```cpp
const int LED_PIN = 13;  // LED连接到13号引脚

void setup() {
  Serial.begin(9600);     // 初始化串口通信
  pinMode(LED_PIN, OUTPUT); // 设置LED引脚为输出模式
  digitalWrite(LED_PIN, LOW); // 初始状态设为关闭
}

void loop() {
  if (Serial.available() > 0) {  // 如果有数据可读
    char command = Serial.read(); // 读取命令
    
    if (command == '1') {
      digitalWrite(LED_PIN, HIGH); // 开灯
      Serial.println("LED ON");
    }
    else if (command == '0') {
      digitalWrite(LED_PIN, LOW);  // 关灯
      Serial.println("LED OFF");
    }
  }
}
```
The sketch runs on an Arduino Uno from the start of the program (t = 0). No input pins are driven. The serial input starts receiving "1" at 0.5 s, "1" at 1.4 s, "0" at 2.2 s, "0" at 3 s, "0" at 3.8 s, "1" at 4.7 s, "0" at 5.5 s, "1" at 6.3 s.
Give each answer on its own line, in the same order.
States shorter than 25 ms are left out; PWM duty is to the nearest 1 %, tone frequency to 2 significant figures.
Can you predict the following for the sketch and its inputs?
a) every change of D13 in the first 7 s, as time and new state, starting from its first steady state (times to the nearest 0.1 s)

0 s low; 0.5 s high; 2.2 s low; 4.7 s high; 5.5 s low; 6.3 s high
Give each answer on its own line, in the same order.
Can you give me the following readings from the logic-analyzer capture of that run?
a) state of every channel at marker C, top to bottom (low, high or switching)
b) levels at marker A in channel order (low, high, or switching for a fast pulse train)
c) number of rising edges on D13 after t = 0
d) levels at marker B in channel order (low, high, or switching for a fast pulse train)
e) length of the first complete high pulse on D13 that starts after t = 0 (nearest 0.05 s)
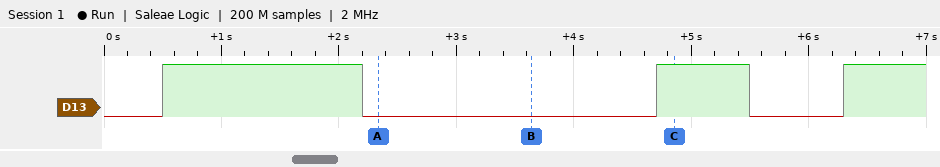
D13 high
D13 low
3
D13 low
1.70 s
